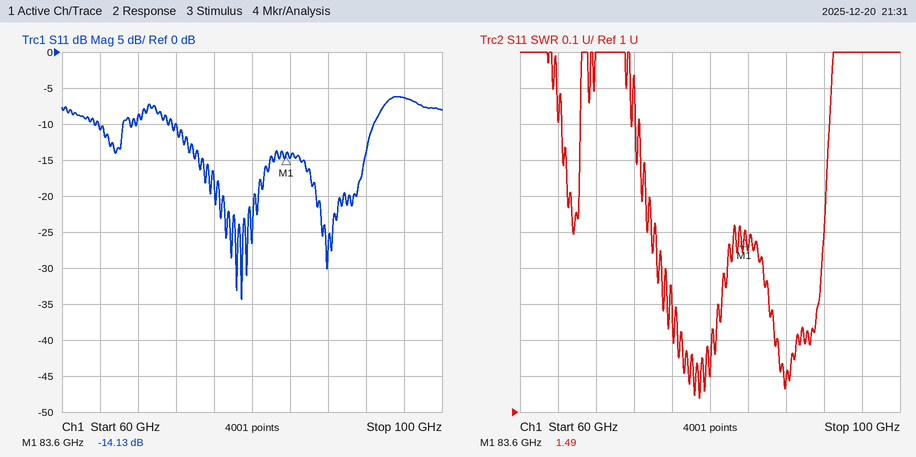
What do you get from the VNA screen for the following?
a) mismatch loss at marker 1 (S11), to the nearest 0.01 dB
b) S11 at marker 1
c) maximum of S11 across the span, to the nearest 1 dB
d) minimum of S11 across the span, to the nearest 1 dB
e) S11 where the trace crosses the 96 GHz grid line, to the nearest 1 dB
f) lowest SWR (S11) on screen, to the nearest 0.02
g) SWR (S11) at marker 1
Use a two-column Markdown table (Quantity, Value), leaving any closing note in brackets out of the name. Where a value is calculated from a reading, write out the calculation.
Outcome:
| Quantity | Value |
|---|---|
| mismatch loss at marker 1 (S11), to the nearest 0.01 dB | −10 log10(1 − 10^(-14.13/10)) ≈ 0.17 dB |
| S11 at marker 1 | -14.13 dB |
| maximum of S11 across the span, to the nearest 1 dB | -6 dB |
| minimum of S11 across the span, to the nearest 1 dB | -34 dB |
| S11 where the trace crosses the 96 GHz grid line, to the nearest 1 dB | -6 dB |
| lowest SWR (S11) on screen, to the nearest 0.02 | 1.04 |
| SWR (S11) at marker 1 | 1.49 |
